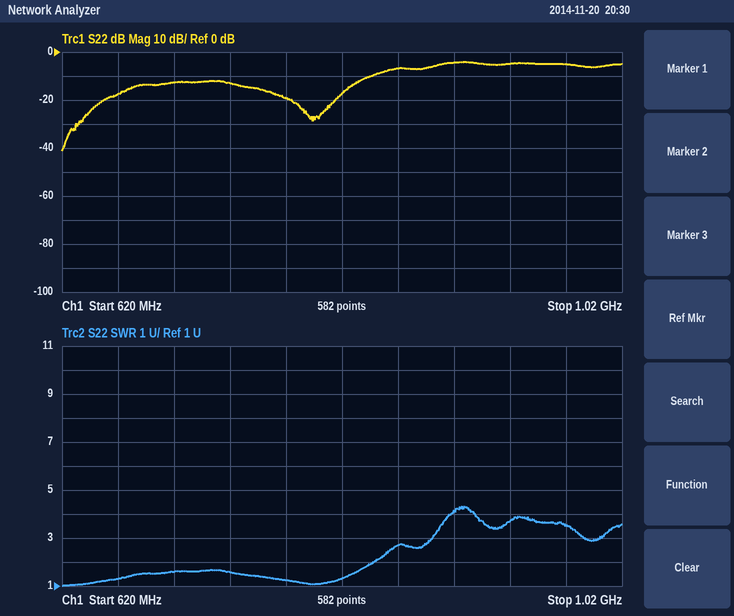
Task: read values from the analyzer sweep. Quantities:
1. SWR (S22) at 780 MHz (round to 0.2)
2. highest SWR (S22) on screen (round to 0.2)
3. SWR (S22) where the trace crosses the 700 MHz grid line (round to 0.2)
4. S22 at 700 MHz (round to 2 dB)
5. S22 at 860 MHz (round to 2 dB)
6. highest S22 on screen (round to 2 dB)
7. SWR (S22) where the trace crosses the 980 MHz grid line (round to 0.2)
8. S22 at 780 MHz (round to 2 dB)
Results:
1.2
4.4
1.6
-12 dB
-6 dB
-4 dB
3.6
-20 dB
